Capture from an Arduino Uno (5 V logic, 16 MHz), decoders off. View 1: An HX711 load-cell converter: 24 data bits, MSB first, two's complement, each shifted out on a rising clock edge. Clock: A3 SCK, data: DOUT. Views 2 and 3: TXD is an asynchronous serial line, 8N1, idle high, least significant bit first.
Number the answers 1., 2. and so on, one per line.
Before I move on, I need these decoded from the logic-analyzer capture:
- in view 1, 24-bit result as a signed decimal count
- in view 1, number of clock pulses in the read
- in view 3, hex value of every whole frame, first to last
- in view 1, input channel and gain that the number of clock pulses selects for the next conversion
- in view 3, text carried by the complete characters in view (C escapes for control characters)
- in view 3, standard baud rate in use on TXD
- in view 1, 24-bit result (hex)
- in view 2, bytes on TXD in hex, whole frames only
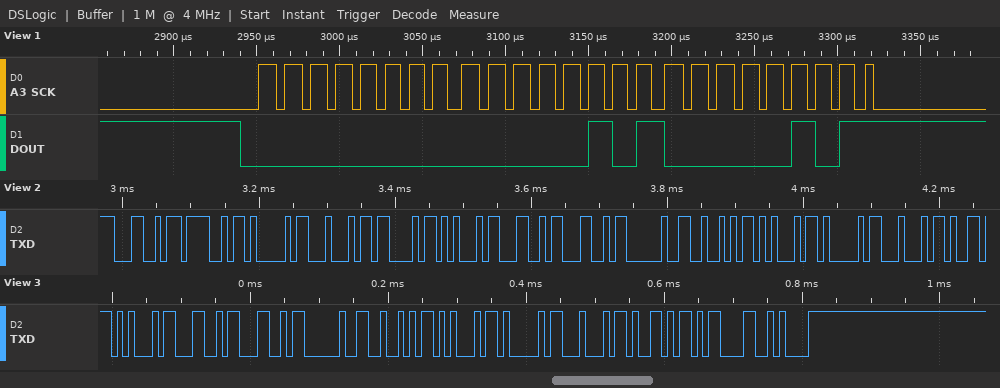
1. 1285
2. 25
3. 0x45 0x4C 0x4C 0x20 0x52 0x45 0x41 0x44 0x59 0x0D 0x0A
4. channel A, gain 128
5. "ELL READY\r\n"
6. 115200 baud
7. 0x000505
8. 4C 4F 41 44 43 45 4C 4C 20 52 45 41 44
